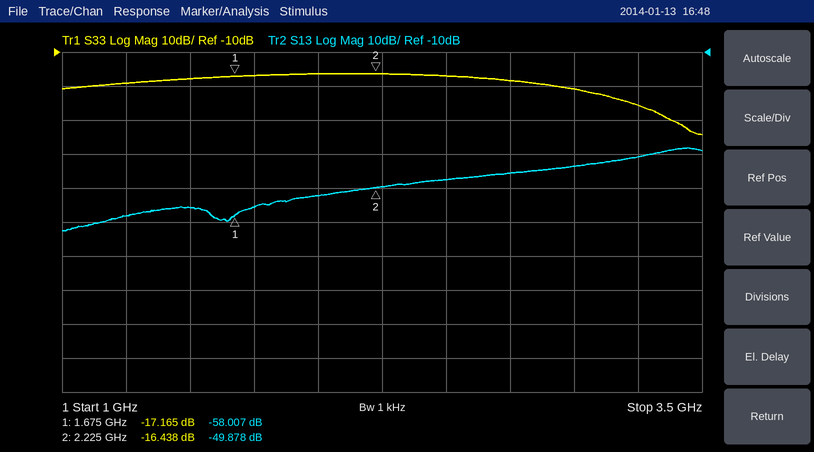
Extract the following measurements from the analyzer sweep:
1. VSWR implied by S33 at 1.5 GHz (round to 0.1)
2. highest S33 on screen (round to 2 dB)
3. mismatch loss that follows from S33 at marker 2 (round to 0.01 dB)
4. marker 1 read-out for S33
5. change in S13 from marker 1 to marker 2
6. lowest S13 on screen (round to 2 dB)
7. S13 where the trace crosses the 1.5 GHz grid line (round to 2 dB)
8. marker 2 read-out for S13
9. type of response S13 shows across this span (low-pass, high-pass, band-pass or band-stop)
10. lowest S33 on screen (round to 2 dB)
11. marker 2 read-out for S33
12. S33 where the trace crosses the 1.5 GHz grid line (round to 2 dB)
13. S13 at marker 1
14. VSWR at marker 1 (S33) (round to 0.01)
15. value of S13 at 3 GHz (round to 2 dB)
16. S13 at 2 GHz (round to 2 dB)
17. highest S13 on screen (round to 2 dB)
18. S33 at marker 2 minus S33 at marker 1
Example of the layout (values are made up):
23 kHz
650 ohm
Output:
1.3
-16 dB
0.10 dB
-17.165 dB
8.129 dB
-62 dB
-56 dB
-49.878 dB
high-pass
-34 dB
-16.438 dB
-18 dB
-58.007 dB
1.32
-44 dB
-52 dB
-38 dB
0.727 dB
